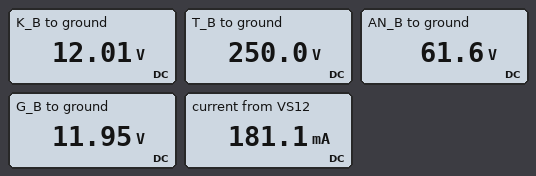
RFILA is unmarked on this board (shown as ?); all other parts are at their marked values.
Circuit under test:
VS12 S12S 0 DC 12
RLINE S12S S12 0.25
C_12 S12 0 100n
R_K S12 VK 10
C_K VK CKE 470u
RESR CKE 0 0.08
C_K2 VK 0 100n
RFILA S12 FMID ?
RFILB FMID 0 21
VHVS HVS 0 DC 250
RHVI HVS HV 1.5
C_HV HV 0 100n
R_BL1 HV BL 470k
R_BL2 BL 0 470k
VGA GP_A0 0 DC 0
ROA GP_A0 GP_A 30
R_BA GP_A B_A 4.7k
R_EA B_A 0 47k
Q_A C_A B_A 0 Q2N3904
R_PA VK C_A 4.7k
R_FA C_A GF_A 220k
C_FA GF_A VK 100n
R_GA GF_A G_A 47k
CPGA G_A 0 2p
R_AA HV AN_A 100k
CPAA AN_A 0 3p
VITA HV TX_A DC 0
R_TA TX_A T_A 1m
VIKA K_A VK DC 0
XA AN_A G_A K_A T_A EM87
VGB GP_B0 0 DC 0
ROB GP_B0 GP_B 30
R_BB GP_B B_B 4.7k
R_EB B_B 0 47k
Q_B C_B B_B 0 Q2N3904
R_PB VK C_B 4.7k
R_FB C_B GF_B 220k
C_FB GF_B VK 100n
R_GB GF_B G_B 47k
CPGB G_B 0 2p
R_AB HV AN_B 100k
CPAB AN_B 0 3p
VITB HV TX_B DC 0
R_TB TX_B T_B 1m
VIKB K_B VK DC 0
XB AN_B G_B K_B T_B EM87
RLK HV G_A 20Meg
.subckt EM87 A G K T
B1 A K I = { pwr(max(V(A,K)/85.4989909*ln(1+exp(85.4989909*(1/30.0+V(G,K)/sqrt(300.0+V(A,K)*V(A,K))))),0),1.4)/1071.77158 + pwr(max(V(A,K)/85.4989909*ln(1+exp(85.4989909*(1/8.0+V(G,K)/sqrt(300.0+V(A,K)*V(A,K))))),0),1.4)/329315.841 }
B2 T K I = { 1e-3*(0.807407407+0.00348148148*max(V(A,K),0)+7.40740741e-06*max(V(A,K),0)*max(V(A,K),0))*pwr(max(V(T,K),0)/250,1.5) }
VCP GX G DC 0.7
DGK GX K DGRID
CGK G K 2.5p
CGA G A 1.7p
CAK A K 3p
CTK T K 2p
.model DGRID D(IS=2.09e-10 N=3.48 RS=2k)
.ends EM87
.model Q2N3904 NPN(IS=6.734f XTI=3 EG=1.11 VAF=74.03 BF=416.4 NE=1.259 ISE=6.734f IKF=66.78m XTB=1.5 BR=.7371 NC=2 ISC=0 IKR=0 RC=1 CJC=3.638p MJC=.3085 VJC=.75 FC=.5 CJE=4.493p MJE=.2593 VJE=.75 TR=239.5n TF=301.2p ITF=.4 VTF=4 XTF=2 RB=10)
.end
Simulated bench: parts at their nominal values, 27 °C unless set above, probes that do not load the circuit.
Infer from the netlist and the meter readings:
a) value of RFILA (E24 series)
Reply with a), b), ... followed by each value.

a) 43 Ω
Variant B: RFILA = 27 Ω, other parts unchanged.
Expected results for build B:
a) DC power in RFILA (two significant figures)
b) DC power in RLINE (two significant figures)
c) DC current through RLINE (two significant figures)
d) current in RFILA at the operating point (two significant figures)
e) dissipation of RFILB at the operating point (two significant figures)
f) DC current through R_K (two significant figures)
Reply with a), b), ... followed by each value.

a) 1.7 W
b) 15 mW
c) 240 mA
d) 250 mA
e) 1.3 W
f) 5.7 mA
